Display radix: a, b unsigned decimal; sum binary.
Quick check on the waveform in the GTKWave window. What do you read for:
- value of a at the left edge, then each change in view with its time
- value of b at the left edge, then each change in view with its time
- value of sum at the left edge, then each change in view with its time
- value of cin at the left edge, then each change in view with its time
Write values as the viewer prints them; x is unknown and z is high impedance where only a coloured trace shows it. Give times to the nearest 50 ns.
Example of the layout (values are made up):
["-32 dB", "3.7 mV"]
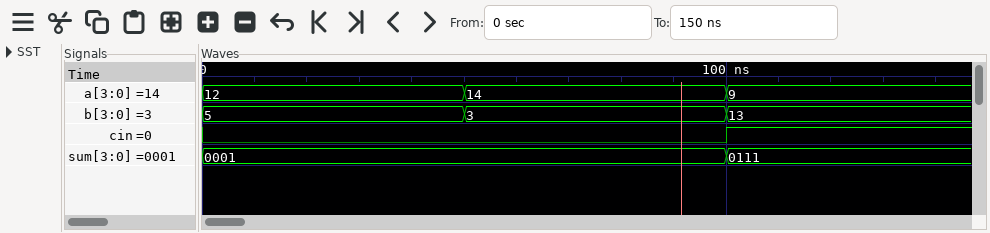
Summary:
["12, 14 at 50 ns, 9 at 100 ns", "5, 3 at 50 ns, 13 at 100 ns", "0001, 0111 at 100 ns", "0, 1 at 100 ns"]
